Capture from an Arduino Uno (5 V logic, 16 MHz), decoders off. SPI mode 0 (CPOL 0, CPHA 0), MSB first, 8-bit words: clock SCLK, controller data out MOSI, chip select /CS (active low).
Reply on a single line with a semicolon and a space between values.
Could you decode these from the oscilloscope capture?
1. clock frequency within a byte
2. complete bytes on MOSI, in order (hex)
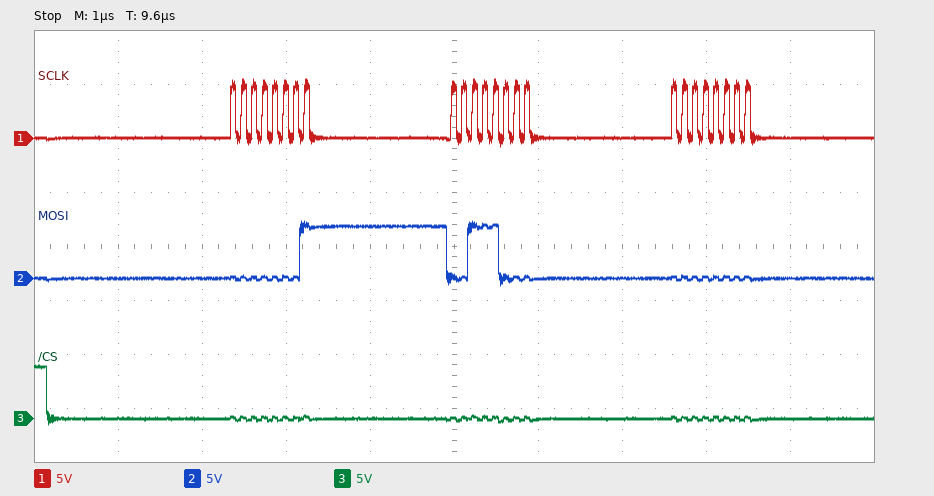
8 MHz; 01 38 00
